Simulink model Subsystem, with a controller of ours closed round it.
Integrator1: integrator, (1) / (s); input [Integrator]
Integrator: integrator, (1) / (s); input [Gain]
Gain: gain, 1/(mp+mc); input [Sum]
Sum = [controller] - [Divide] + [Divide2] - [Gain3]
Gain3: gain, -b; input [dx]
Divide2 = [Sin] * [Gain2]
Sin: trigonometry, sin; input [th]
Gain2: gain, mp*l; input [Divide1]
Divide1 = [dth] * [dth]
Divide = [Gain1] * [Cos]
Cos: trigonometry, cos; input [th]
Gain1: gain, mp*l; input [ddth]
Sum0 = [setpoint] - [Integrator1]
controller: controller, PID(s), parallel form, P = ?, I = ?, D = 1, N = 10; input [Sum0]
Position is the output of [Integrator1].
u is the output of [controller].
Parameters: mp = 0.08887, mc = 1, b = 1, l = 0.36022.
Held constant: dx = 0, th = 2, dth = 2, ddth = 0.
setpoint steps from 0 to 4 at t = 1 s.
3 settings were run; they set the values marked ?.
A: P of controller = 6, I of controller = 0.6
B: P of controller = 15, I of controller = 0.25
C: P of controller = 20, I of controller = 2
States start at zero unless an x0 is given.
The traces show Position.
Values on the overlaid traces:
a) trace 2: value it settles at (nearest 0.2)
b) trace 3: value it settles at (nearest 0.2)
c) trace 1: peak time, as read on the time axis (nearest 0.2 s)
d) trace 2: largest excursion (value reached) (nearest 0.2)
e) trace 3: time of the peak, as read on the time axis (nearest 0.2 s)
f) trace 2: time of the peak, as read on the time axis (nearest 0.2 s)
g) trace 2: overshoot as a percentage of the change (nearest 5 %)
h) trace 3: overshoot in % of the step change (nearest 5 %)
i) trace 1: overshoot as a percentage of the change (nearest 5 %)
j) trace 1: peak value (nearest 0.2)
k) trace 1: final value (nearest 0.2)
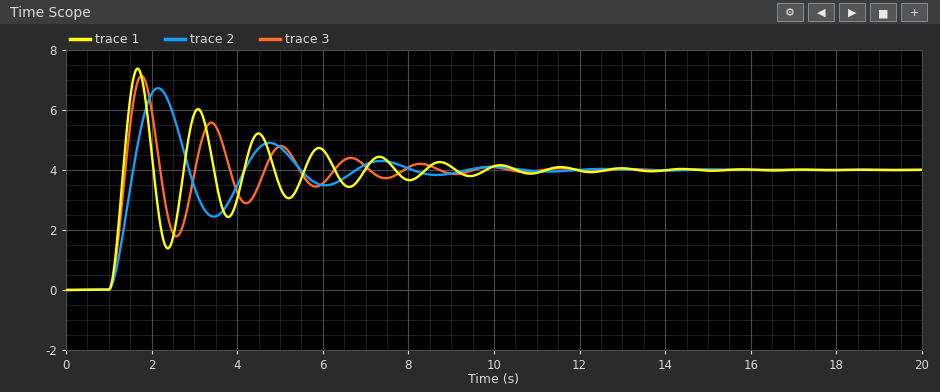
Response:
4.0
4.0
1.6 s
6.8
1.8 s
2.2 s
70 %
80 %
85 %
7.4
4.0
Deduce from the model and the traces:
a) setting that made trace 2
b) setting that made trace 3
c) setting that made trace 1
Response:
A
B
C
